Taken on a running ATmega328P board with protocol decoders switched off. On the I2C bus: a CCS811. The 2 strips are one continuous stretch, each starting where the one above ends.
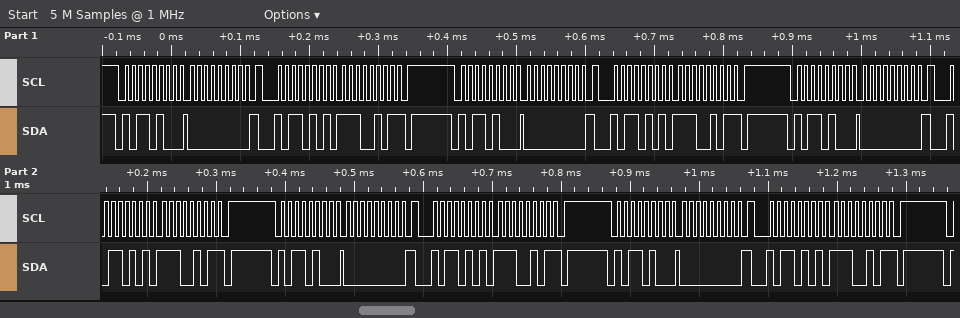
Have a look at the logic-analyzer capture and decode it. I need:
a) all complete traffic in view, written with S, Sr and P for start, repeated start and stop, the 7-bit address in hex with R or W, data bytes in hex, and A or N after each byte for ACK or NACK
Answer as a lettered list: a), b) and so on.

a) S 5AW A 00 A Sr 5AR A E5 N P S 5AW A 00 A Sr 5AR A E5 N P S 5AW A 00 A Sr 5AR A E5 N P S 5AW A 00 A Sr 5AR A E5 N P S 5AW A 00 A Sr 5AR A E5 N P
